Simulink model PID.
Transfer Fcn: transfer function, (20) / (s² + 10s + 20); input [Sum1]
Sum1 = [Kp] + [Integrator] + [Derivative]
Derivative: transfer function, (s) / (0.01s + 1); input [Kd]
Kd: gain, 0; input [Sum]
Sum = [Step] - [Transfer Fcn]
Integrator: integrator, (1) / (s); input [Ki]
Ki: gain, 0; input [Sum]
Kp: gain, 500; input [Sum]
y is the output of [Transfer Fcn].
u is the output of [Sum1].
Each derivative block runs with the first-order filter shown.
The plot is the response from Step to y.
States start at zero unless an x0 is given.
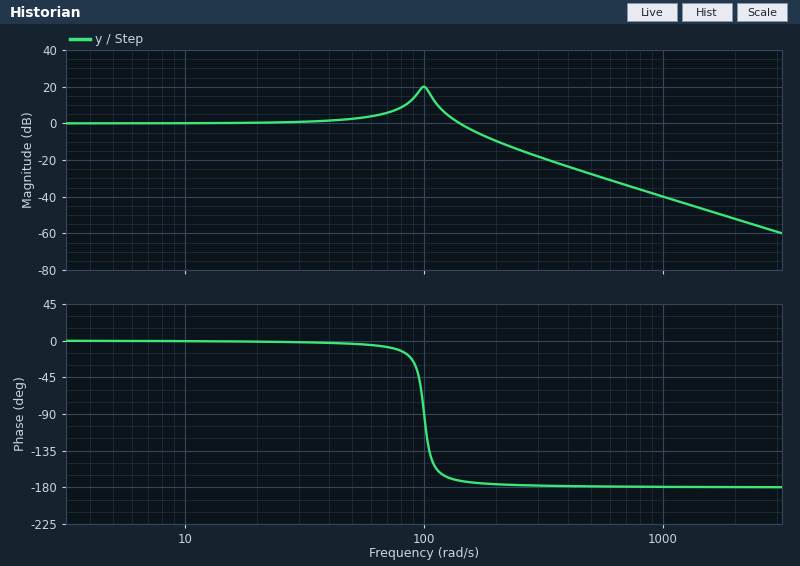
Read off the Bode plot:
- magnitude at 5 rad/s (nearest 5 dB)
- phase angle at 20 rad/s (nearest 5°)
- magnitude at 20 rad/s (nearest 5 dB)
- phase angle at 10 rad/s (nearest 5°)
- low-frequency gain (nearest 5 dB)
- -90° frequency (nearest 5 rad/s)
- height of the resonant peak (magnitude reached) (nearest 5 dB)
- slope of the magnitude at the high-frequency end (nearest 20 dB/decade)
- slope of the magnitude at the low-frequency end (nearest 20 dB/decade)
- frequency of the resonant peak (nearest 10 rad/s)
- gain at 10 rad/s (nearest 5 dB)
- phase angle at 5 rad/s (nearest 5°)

0 dB
0°
0 dB
0°
0 dB
100 rad/s
20 dB
-40 dB/decade
0 dB/decade
100 rad/s
0 dB
0°
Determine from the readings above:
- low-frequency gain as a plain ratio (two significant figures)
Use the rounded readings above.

1.0
